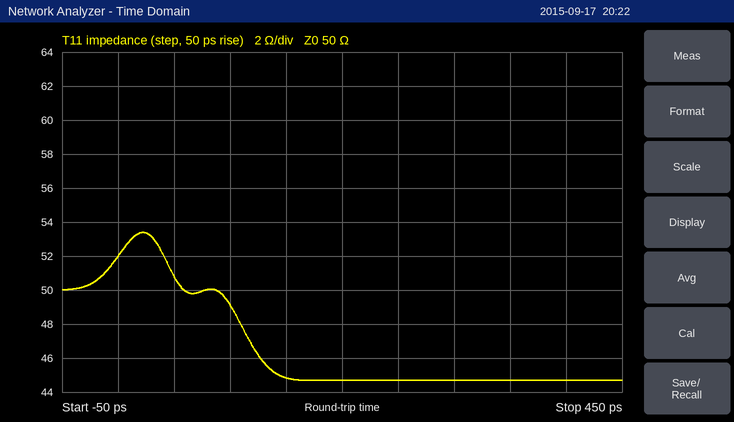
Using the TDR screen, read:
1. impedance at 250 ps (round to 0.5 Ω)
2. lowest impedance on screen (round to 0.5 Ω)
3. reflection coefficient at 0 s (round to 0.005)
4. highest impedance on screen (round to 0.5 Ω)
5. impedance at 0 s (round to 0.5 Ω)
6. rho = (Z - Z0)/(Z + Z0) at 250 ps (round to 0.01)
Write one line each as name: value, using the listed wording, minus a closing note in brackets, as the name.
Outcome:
impedance at 250 ps: 44.5 Ω
lowest impedance on screen: 44.5 Ω
reflection coefficient at 0 s: +0.020
highest impedance on screen: 53.5 Ω
impedance at 0 s: 52.0 Ω
rho = (Z - Z0)/(Z + Z0) at 250 ps: -0.06
